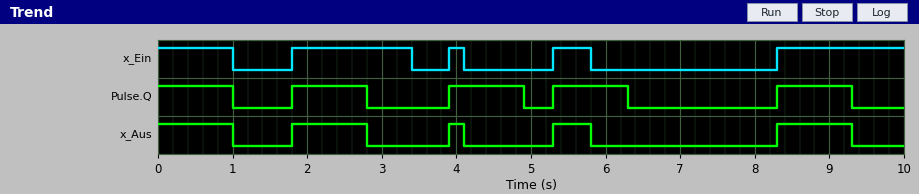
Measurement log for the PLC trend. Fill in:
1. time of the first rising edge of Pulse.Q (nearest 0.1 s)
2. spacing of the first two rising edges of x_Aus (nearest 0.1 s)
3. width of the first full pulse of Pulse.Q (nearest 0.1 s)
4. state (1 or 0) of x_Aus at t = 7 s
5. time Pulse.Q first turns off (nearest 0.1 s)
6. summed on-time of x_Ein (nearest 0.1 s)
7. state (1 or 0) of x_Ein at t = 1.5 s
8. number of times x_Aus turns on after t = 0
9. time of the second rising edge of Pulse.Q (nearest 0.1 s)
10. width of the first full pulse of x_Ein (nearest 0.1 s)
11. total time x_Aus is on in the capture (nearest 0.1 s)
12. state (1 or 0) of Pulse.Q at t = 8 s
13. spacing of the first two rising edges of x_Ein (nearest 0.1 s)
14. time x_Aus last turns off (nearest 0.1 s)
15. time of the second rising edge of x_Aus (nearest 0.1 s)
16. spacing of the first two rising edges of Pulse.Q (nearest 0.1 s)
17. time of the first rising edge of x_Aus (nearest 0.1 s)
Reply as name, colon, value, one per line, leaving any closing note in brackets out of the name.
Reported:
time of the first rising edge of Pulse.Q: 1.8 s
spacing of the first two rising edges of x_Aus: 2.1 s
width of the first full pulse of Pulse.Q: 1.0 s
state (1 or 0) of x_Aus at t = 7 s: 0
time Pulse.Q first turns off: 1.0 s
summed on-time of x_Ein: 5.0 s
state (1 or 0) of x_Ein at t = 1.5 s: 0
number of times x_Aus turns on after t = 0: 4
time of the second rising edge of Pulse.Q: 3.9 s
width of the first full pulse of x_Ein: 1.6 s
total time x_Aus is on in the capture: 3.7 s
state (1 or 0) of Pulse.Q at t = 8 s: 0
spacing of the first two rising edges of x_Ein: 2.1 s
time x_Aus last turns off: 9.3 s
time of the second rising edge of x_Aus: 3.9 s
spacing of the first two rising edges of Pulse.Q: 2.1 s
time of the first rising edge of x_Aus: 1.8 s
